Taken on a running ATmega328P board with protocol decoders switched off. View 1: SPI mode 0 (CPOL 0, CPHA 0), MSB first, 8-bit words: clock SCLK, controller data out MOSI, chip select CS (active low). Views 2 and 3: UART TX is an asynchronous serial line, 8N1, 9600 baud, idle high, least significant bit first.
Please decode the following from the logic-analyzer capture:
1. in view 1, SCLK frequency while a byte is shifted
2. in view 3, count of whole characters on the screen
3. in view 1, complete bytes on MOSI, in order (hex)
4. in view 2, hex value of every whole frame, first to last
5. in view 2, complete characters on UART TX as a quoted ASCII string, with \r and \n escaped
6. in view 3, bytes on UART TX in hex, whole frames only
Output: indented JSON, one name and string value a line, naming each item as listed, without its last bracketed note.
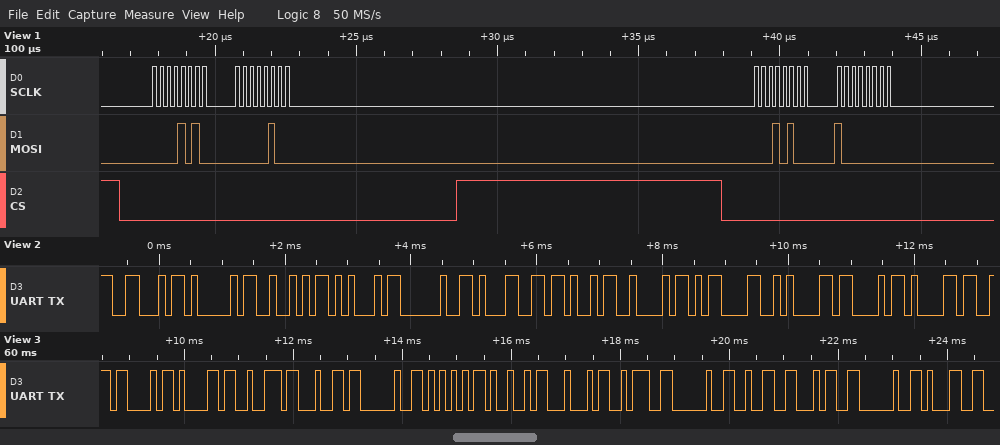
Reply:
{
  "in view 1, SCLK frequency while a byte is shifted": "4 MHz",
  "in view 3, count of whole characters on the screen": "14",
  "in view 1, complete bytes on MOSI, in order": "0A 04 14 80",
  "in view 2, hex value of every whole frame, first to last": "0x46 0x41 0x52 0x45 0x20 0x31 0x4B 0x42 0x0D 0x0A 0x43 0x61",
  "in view 2, complete characters on UART TX as a quoted ASCII string, with \\r and \\n escaped": "\"FARE 1KB\\r\\nCa\"",
  "in view 3, bytes on UART TX in hex, whole frames only": "43 61 72 64 20 55 49 44 3A 20 32 34 20 31"
}
